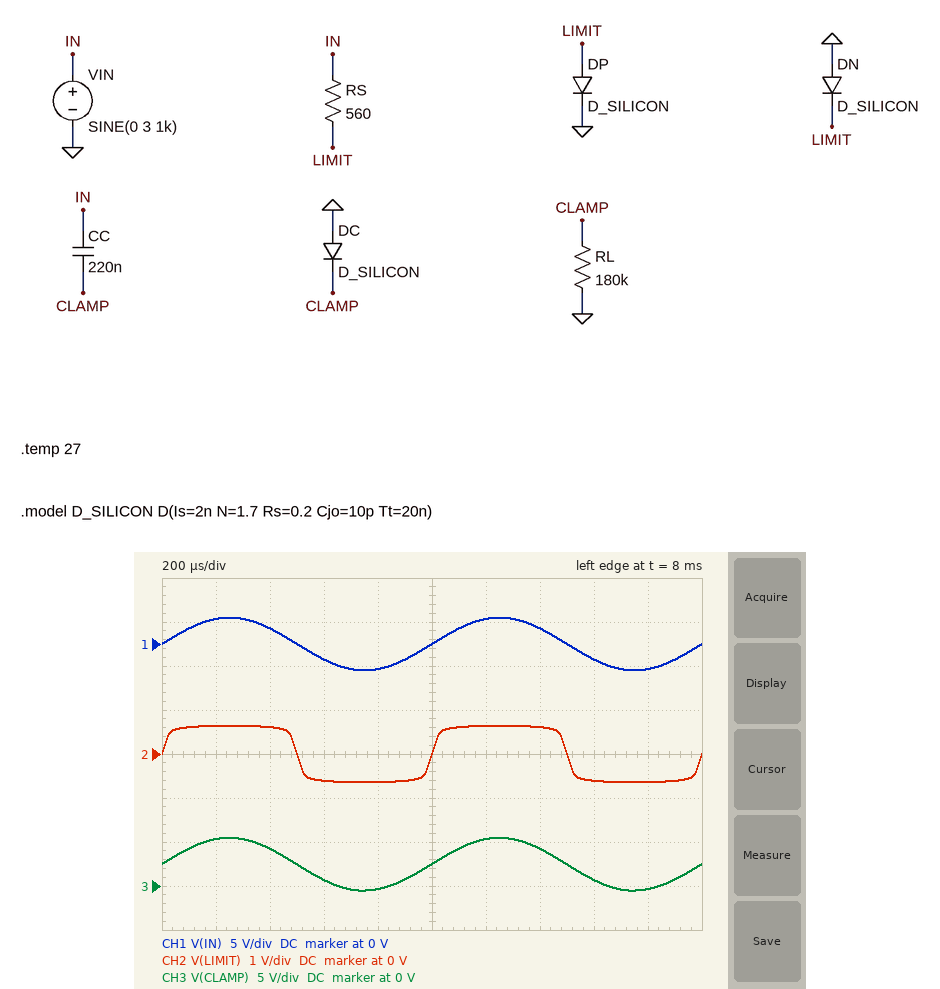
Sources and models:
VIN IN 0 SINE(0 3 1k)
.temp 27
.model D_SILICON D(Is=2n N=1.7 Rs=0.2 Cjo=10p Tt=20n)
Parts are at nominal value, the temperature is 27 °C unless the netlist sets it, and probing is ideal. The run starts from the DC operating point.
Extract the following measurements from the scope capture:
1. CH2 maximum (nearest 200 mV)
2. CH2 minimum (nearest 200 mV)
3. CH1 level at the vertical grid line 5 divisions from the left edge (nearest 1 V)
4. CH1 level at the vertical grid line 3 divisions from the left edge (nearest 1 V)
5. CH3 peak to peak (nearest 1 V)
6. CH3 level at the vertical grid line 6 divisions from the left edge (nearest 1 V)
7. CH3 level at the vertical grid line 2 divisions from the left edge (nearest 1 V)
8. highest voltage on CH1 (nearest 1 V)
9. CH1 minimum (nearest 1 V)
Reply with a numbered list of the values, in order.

1. 600 mV
2. -600 mV
3. 0 V
4. -2 V
5. 6 V
6. 5 V
7. 4 V
8. 3 V
9. -3 V
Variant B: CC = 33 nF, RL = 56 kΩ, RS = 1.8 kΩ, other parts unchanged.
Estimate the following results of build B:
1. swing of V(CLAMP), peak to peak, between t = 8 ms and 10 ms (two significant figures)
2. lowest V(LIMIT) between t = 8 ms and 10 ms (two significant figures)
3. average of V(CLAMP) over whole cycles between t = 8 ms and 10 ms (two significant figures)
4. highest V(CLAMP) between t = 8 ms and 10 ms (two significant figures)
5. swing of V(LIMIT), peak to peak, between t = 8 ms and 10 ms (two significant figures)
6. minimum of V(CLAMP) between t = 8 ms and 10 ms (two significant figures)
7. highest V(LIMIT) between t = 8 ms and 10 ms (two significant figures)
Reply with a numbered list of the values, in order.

1. 5.5 V
2. -590 mV
3. 2.1 V
4. 5.0 V
5. 1.2 V
6. -540 mV
7. 590 mV
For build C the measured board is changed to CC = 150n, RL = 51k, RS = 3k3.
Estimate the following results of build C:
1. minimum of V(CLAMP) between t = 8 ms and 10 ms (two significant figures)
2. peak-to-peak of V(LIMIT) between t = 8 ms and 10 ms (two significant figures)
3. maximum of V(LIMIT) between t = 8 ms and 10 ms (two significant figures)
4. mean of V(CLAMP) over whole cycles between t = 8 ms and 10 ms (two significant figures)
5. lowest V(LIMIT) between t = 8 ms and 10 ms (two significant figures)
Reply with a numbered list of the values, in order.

1. -570 mV
2. 1.1 V
3. 560 mV
4. 2.4 V
5. -560 mV
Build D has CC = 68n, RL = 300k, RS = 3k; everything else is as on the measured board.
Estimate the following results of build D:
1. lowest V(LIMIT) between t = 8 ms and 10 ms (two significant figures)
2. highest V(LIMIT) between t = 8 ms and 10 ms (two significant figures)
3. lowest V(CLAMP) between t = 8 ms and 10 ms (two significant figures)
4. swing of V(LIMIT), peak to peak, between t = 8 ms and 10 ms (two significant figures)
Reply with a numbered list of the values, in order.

1. -570 mV
2. 570 mV
3. -500 mV
4. 1.1 V
